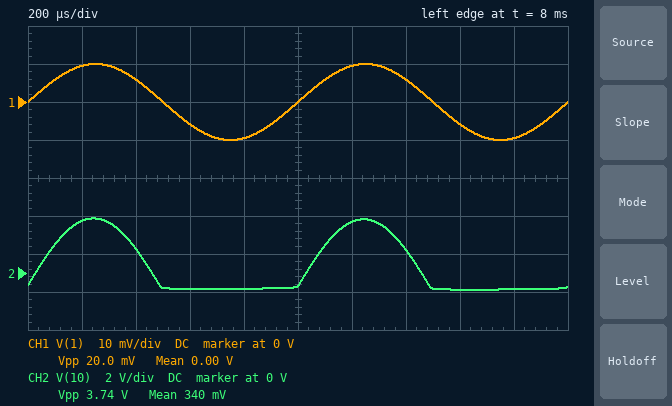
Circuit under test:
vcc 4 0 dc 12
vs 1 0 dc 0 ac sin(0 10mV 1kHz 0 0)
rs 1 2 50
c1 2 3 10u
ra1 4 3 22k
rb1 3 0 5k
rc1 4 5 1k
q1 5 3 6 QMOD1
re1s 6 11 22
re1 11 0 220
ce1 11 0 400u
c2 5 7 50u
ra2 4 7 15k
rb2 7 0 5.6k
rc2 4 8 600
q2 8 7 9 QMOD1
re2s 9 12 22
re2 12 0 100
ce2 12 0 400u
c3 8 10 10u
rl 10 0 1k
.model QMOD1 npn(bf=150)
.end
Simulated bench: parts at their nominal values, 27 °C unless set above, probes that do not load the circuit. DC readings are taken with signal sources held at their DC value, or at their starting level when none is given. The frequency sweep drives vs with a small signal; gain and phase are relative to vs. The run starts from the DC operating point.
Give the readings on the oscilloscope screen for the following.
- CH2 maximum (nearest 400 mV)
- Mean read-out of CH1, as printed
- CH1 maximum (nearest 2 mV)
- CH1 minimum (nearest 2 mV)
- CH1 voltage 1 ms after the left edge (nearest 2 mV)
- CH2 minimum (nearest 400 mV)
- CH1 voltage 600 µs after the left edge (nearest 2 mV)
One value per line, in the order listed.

2.8 V
0.00 V
10 mV
-10 mV
0 V
-800 mV
-6 mV
